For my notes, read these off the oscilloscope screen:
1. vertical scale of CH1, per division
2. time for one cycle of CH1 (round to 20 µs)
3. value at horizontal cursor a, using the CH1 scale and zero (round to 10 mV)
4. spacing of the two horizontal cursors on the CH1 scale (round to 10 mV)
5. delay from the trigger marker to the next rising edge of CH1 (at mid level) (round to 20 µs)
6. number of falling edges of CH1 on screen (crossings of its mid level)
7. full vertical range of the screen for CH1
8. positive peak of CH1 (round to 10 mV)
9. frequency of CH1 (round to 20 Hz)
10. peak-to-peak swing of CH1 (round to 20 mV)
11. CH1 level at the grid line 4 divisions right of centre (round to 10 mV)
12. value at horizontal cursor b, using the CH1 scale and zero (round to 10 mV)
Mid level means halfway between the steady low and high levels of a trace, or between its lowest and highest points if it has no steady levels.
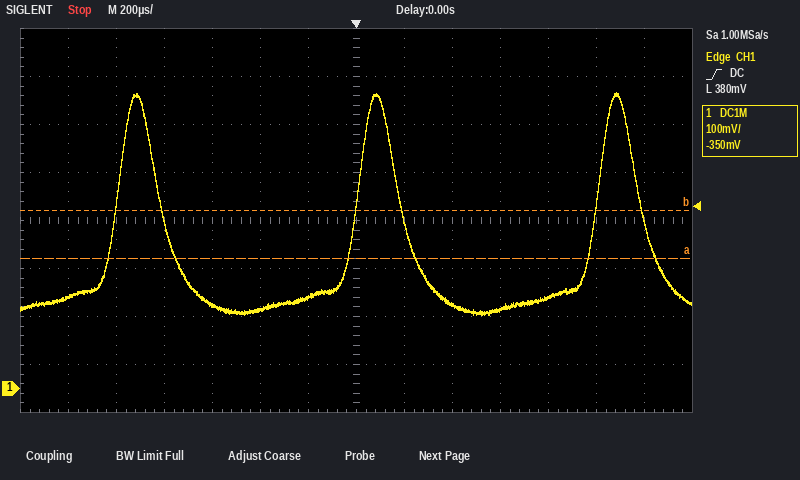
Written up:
100 mV
1.00 ms
270 mV
100 mV
1.00 ms
3
800 mV
620 mV
1.00 kHz
460 mV
190 mV
370 mV
